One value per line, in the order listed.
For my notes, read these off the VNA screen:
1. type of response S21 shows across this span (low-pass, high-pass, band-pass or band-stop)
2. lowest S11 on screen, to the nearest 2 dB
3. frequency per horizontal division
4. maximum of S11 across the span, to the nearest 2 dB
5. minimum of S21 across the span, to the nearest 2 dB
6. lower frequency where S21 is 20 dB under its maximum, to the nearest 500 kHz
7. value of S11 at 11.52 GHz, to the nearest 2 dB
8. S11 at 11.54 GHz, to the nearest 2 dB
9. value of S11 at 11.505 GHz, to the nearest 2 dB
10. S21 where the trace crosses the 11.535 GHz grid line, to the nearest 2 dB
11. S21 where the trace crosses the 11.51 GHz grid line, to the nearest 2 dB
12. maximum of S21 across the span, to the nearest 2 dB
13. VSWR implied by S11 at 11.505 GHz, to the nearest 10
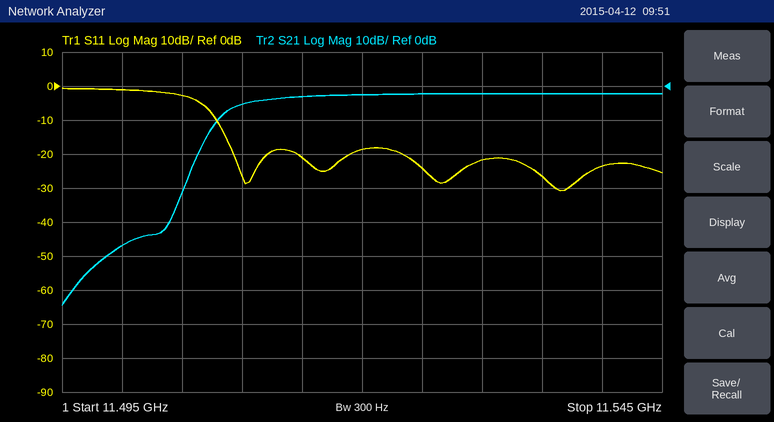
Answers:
high-pass
-30 dB
5 MHz
0 dB
-64 dB
11.5060 GHz
-18 dB
-24 dB
-2 dB
-2 dB
-6 dB
-2 dB
10
